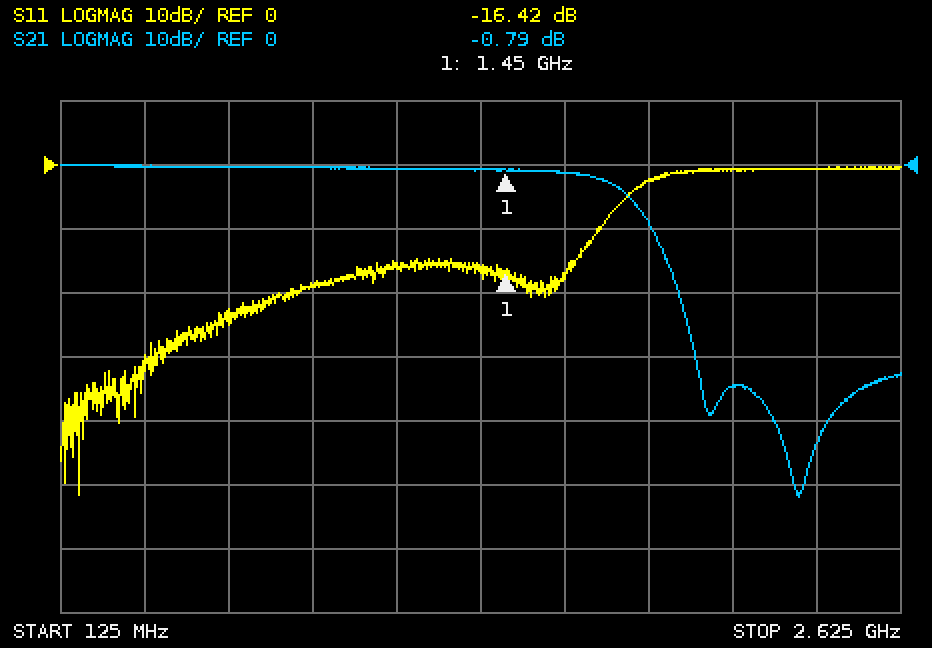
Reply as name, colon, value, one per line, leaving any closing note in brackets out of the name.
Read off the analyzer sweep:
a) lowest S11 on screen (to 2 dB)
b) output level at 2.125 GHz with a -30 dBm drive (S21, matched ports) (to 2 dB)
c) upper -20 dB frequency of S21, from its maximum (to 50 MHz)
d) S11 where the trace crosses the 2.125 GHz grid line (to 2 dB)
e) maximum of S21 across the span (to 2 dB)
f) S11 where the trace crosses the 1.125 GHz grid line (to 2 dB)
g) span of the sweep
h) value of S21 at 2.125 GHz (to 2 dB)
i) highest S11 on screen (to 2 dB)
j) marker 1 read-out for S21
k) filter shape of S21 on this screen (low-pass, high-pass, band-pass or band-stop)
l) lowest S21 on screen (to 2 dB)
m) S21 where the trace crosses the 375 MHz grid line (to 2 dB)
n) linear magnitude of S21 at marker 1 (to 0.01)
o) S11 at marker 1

lowest S11 on screen: -52 dB
output level at 2.125 GHz with a -30 dBm drive (S21, matched ports): -64 dBm
upper -20 dB frequency of S21, from its maximum: 1.95 GHz
S11 where the trace crosses the 2.125 GHz grid line: 0 dB
maximum of S21 across the span: 0 dB
S11 where the trace crosses the 1.125 GHz grid line: -16 dB
span of the sweep: 2.5 GHz
value of S21 at 2.125 GHz: -34 dB
highest S11 on screen: 0 dB
marker 1 read-out for S21: -0.79 dB
filter shape of S21 on this screen: low-pass
lowest S21 on screen: -52 dB
S21 where the trace crosses the 375 MHz grid line: 0 dB
linear magnitude of S21 at marker 1: 0.91
S11 at marker 1: -16.42 dB
